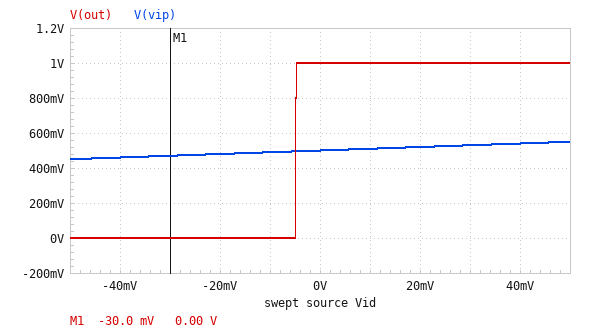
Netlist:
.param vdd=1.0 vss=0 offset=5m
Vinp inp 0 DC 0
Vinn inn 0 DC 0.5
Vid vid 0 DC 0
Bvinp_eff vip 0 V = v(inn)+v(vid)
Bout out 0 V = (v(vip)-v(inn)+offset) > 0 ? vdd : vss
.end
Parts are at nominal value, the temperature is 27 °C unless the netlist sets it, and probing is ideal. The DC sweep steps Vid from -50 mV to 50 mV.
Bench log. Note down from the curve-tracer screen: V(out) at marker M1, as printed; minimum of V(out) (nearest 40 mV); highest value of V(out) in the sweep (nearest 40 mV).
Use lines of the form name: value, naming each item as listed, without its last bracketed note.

V(out) at marker M1, as printed: 0.00 V
minimum of V(out): 0 V
highest value of V(out) in the sweep: 1.00 V
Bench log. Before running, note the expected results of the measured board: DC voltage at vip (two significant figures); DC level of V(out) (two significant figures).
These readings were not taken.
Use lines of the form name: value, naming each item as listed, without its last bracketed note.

DC voltage at vip: 500 mV
DC level of V(out): 1.0 V
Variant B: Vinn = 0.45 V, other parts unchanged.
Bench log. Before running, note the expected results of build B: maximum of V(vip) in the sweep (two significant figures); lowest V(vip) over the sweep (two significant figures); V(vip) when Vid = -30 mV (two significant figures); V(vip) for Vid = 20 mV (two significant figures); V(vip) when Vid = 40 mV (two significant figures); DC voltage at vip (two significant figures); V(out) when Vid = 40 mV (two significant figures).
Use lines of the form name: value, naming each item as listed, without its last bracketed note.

maximum of V(vip) in the sweep: 500 mV
lowest V(vip) over the sweep: 400 mV
V(vip) when Vid = -30 mV: 420 mV
V(vip) for Vid = 20 mV: 470 mV
V(vip) when Vid = 40 mV: 490 mV
DC voltage at vip: 450 mV
V(out) when Vid = 40 mV: 1.0 V
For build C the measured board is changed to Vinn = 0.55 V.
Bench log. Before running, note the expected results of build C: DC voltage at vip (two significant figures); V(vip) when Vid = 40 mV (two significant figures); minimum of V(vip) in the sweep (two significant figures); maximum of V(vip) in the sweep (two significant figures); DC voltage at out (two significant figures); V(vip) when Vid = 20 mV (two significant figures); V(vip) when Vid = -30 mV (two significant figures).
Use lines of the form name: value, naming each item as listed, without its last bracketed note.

DC voltage at vip: 550 mV
V(vip) when Vid = 40 mV: 590 mV
minimum of V(vip) in the sweep: 500 mV
maximum of V(vip) in the sweep: 600 mV
DC voltage at out: 1.0 V
V(vip) when Vid = 20 mV: 570 mV
V(vip) when Vid = -30 mV: 520 mV
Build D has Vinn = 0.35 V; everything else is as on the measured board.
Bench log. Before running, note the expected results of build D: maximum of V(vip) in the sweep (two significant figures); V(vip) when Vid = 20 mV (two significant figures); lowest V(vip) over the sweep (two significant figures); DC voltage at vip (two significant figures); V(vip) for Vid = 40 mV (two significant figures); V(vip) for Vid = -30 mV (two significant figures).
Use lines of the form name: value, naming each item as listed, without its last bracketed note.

maximum of V(vip) in the sweep: 400 mV
V(vip) when Vid = 20 mV: 370 mV
lowest V(vip) over the sweep: 300 mV
DC voltage at vip: 350 mV
V(vip) for Vid = 40 mV: 390 mV
V(vip) for Vid = -30 mV: 320 mV
